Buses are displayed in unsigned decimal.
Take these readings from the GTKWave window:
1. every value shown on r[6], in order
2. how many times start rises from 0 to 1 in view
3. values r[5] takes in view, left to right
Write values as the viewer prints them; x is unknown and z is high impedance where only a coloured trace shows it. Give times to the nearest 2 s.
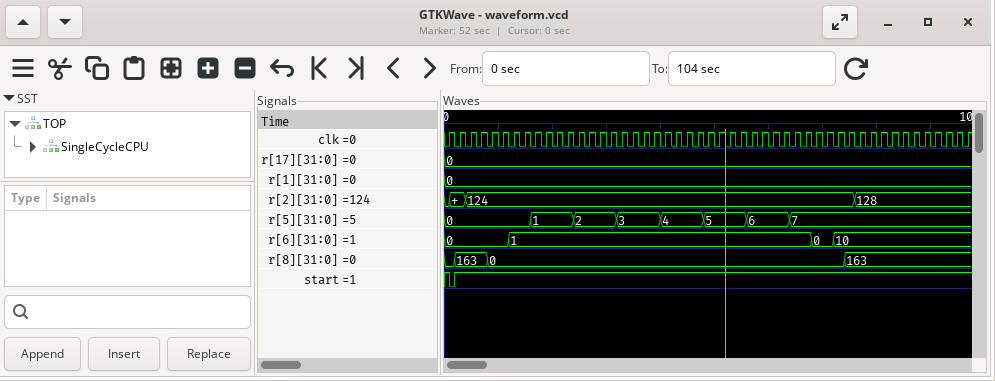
0, 1, 0, 10
1
0, 1, 2, 3, 4, 5, 6, 7
